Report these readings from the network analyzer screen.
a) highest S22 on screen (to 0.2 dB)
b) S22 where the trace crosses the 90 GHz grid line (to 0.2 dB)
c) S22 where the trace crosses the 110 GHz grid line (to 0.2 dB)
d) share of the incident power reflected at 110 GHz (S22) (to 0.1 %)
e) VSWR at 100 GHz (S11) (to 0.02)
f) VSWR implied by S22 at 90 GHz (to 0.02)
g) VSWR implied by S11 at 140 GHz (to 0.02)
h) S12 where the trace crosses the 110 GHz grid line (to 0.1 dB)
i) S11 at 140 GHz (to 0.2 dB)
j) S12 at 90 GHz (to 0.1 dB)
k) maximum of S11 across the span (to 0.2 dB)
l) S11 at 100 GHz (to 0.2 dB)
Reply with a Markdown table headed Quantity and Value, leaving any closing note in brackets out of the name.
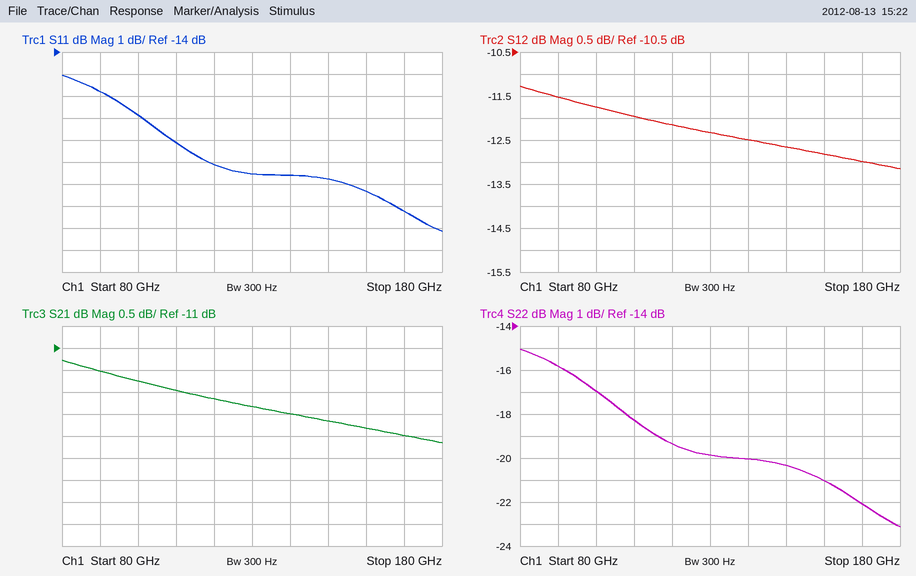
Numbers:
| Quantity | Value |
|---|---|
| highest S22 on screen | -15.0 dB |
| S22 where the trace crosses the 90 GHz grid line | -15.8 dB |
| S22 where the trace crosses the 110 GHz grid line | -18.2 dB |
| share of the incident power reflected at 110 GHz (S22) | 1.5 % |
| VSWR at 100 GHz (S11) | 1.34 |
| VSWR implied by S22 at 90 GHz | 1.38 |
| VSWR implied by S11 at 140 GHz | 1.24 |
| S12 where the trace crosses the 110 GHz grid line | -12.0 dB |
| S11 at 140 GHz | -19.6 dB |
| S12 at 90 GHz | -11.5 dB |
| maximum of S11 across the span | -15.0 dB |
| S11 at 100 GHz | -16.8 dB |
